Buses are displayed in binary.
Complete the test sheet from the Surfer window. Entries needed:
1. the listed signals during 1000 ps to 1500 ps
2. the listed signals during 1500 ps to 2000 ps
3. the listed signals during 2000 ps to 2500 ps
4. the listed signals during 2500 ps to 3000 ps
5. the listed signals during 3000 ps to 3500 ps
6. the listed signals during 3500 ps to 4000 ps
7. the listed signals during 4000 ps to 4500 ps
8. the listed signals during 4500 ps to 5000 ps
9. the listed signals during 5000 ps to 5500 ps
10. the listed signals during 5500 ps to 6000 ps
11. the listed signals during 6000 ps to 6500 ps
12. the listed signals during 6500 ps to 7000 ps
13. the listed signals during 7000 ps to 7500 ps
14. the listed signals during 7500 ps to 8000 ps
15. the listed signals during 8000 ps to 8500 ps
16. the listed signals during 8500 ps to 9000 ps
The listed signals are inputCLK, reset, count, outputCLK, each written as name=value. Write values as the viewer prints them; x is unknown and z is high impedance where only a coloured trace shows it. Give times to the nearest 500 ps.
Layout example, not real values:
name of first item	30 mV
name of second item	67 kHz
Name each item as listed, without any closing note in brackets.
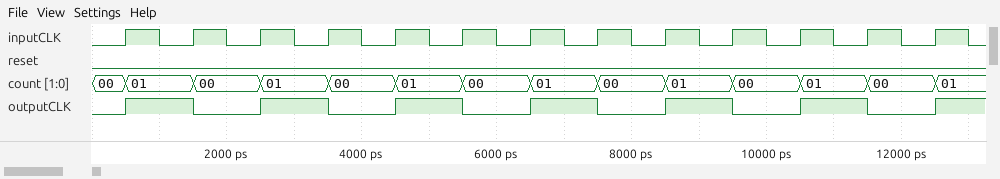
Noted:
the listed signals during 1000 ps to 1500 ps	inputCLK=0, reset=0, count=01, outputCLK=1
the listed signals during 1500 ps to 2000 ps	inputCLK=1, reset=0, count=00, outputCLK=0
the listed signals during 2000 ps to 2500 ps	inputCLK=0, reset=0, count=00, outputCLK=0
the listed signals during 2500 ps to 3000 ps	inputCLK=1, reset=0, count=01, outputCLK=1
the listed signals during 3000 ps to 3500 ps	inputCLK=0, reset=0, count=01, outputCLK=1
the listed signals during 3500 ps to 4000 ps	inputCLK=1, reset=0, count=00, outputCLK=0
the listed signals during 4000 ps to 4500 ps	inputCLK=0, reset=0, count=00, outputCLK=0
the listed signals during 4500 ps to 5000 ps	inputCLK=1, reset=0, count=01, outputCLK=1
the listed signals during 5000 ps to 5500 ps	inputCLK=0, reset=0, count=01, outputCLK=1
the listed signals during 5500 ps to 6000 ps	inputCLK=1, reset=0, count=00, outputCLK=0
the listed signals during 6000 ps to 6500 ps	inputCLK=0, reset=0, count=00, outputCLK=0
the listed signals during 6500 ps to 7000 ps	inputCLK=1, reset=0, count=01, outputCLK=1
the listed signals during 7000 ps to 7500 ps	inputCLK=0, reset=0, count=01, outputCLK=1
the listed signals during 7500 ps to 8000 ps	inputCLK=1, reset=0, count=00, outputCLK=0
the listed signals during 8000 ps to 8500 ps	inputCLK=0, reset=0, count=00, outputCLK=0
the listed signals during 8500 ps to 9000 ps	inputCLK=1, reset=0, count=01, outputCLK=1
